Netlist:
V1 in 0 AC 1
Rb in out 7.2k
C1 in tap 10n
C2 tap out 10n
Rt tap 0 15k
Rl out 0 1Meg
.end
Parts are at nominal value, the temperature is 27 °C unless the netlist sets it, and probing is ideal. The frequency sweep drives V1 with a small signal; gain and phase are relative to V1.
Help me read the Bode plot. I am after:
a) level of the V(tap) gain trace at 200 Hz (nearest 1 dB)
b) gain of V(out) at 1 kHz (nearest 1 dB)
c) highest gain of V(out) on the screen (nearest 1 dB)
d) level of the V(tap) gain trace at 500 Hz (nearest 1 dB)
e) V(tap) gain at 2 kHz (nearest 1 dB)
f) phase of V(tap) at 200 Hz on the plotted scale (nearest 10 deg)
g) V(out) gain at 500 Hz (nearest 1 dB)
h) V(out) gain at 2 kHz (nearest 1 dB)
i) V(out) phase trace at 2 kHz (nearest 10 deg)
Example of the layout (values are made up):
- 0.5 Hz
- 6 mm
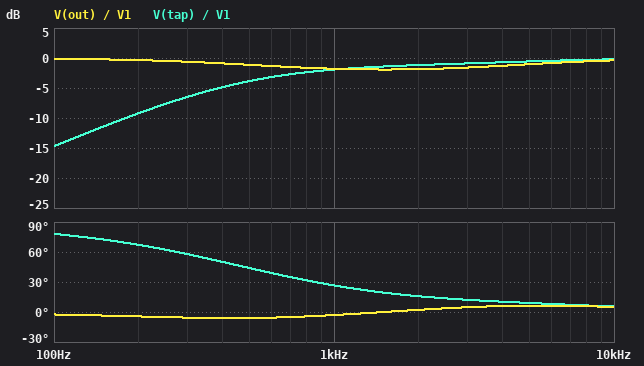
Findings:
- -9 dB
- -2 dB
- 0 dB
- -4 dB
- -1 dB
- 70 deg
- -1 dB
- -2 dB
- 0 deg
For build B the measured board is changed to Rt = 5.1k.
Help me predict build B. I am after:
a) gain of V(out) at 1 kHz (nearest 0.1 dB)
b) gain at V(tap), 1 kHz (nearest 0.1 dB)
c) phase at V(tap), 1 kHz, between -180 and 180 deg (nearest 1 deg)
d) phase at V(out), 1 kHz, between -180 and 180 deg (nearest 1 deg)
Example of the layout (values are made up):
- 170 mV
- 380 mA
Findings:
- -2.3 dB
- -6.5 dB
- 51 deg
- -15 deg
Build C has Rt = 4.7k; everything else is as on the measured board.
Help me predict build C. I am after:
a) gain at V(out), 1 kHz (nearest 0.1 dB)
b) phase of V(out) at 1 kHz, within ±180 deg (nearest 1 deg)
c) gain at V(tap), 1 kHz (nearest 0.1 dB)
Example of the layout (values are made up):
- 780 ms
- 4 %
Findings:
- -2.3 dB
- -16 deg
- -7.0 dB
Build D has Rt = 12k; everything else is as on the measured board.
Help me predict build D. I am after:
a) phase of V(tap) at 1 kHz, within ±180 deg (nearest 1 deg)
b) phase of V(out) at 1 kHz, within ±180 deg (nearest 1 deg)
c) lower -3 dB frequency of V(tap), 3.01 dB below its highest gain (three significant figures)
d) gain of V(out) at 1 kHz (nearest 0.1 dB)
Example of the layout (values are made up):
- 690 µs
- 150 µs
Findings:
- 31 deg
- -5 deg
- 833 Hz
- -2.0 dB
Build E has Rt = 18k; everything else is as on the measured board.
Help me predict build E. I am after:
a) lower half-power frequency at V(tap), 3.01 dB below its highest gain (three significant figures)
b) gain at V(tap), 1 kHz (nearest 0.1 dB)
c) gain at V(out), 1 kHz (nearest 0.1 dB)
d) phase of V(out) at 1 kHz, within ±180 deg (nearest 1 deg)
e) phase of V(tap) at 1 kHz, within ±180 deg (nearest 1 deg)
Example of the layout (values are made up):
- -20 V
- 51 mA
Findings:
- 507 Hz
- -1.5 dB
- -1.6 dB
- -2 deg
- 23 deg
